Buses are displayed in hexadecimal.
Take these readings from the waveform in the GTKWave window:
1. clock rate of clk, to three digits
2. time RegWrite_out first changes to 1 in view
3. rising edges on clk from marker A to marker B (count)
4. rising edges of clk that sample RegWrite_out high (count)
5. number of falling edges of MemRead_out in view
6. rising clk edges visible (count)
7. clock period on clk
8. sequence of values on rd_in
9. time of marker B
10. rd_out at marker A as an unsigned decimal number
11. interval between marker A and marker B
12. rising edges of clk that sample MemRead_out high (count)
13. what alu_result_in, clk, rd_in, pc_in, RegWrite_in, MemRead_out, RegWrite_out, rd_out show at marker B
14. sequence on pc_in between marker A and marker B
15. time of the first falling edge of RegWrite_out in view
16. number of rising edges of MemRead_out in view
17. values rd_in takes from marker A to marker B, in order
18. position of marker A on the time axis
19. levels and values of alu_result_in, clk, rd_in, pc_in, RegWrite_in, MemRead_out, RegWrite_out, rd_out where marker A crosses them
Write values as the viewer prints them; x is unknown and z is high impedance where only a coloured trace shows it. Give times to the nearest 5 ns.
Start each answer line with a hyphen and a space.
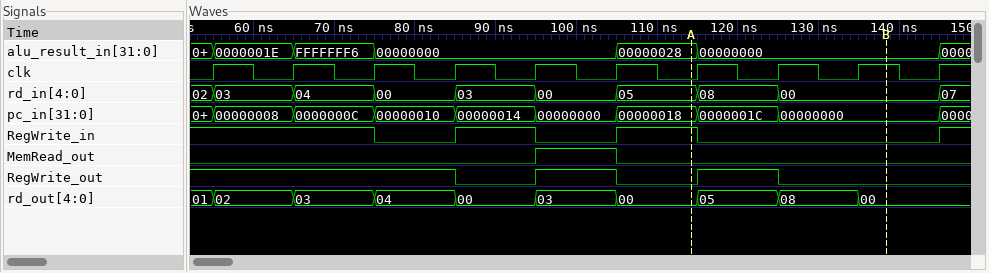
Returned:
- 100 MHz
- 95 ns
- 3
- 6
- 1
- 10
- 10 ns
- 02, 03, 04, 00, 03, 00, 05, 08, 00, 07
- 140 ns
- 0
- 25 ns
- 1
- alu_result_in=00000000, clk=1, rd_in=00, pc_in=00000000, RegWrite_in=0, MemRead_out=0, RegWrite_out=0, rd_out=00
- 00000018, 0000001C, 00000000
- 85 ns
- 1
- 05, 08, 00
- 115 ns
- alu_result_in=00000028, clk=0, rd_in=05, pc_in=00000018, RegWrite_in=1, MemRead_out=0, RegWrite_out=0, rd_out=00
